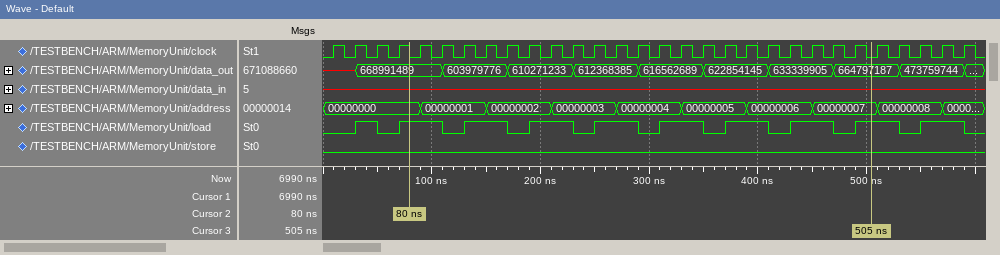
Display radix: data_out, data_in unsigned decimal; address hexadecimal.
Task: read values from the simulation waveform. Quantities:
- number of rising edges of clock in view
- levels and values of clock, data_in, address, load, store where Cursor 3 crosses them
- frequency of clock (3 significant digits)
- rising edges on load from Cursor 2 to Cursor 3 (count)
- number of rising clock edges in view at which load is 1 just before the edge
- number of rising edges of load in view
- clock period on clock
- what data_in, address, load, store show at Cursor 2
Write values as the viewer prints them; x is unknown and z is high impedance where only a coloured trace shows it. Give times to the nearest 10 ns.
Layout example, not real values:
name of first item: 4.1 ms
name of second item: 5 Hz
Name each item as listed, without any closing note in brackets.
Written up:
number of rising edges of clock in view: 30
levels and values of clock, data_in, address, load, store where Cursor 3 crosses them: clock=0, data_in=x, address=00000007, load=1, store=0
frequency of clock: 50.0 MHz
rising edges on load from Cursor 2 to Cursor 3: 7
number of rising clock edges in view at which load is 1 just before the edge: 19
number of rising edges of load in view: 10
clock period on clock: 20 ns
what data_in, address, load, store show at Cursor 2: data_in=x, address=00000000, load=1, store=0
